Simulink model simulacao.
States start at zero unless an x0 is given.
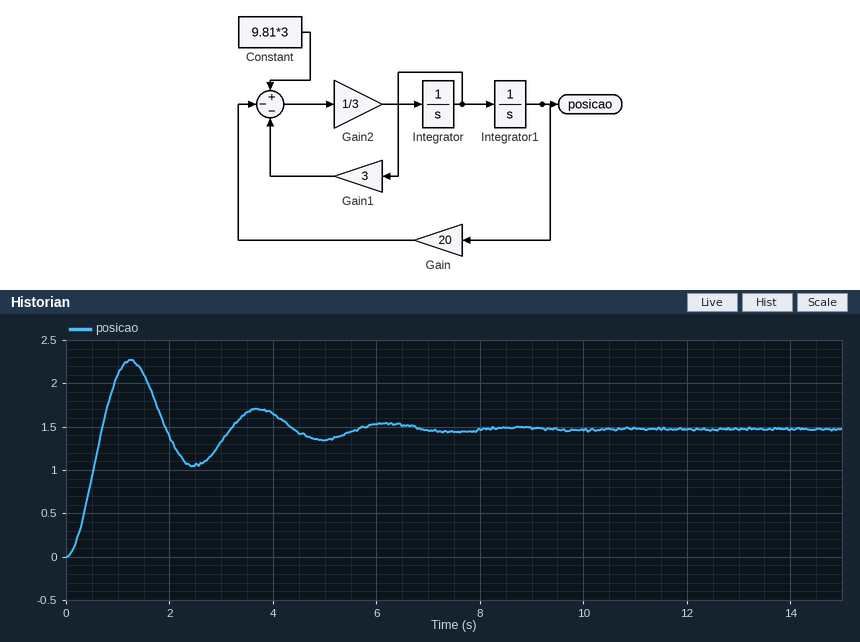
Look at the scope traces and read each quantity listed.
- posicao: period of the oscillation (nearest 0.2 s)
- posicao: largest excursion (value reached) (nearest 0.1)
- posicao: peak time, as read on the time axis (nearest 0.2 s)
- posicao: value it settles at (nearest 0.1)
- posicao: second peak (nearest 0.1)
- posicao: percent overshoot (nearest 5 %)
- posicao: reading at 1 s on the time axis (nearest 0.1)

2.4 s
2.3
1.2 s
1.5
1.7
55 %
2.1
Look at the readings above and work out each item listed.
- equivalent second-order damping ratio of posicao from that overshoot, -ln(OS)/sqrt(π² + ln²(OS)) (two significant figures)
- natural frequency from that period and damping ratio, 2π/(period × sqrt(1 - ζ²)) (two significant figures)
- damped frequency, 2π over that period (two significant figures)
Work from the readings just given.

0.19
2.7 rad/s
2.6 rad/s
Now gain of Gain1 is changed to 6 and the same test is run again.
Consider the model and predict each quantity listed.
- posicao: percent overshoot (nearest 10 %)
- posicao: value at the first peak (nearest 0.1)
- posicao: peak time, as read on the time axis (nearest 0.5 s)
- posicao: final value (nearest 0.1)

30 %
1.9
1.5 s
1.5
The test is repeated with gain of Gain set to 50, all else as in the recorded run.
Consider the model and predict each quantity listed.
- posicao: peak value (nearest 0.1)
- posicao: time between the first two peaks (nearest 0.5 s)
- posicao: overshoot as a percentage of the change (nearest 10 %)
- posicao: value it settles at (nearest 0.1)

1.0
1.5 s
70 %
0.6
